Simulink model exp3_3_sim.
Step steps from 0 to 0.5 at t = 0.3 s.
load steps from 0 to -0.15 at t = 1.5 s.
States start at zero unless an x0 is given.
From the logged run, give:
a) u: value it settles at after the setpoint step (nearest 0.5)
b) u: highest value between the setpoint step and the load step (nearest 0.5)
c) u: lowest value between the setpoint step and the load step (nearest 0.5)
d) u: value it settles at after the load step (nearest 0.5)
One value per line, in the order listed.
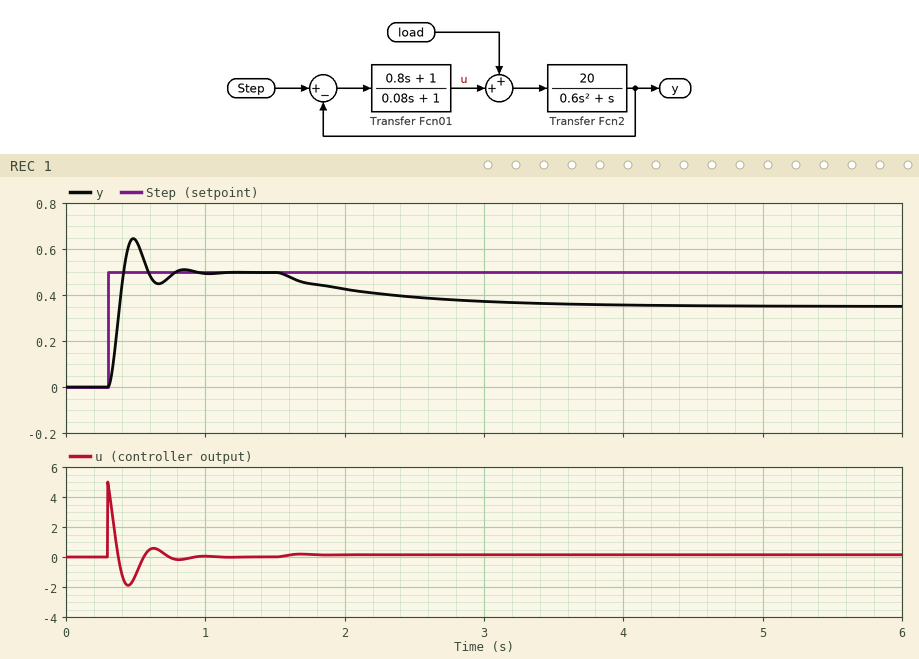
0.0
5.0
-2.0
0.0
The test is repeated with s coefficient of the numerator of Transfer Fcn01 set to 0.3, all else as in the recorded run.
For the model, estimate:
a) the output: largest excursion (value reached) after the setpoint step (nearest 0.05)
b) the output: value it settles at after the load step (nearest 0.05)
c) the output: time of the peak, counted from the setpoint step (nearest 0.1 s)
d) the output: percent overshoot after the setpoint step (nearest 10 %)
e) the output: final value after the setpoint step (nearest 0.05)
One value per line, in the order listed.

0.65
0.35
0.3 s
30 %
0.50
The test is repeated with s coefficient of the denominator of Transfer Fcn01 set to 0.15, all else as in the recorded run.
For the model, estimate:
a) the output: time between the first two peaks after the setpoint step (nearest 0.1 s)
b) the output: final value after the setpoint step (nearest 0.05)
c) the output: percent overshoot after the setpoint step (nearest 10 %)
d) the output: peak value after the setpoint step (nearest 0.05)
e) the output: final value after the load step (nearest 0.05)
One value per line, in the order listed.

0.5 s
0.50
40 %
0.70
0.35
